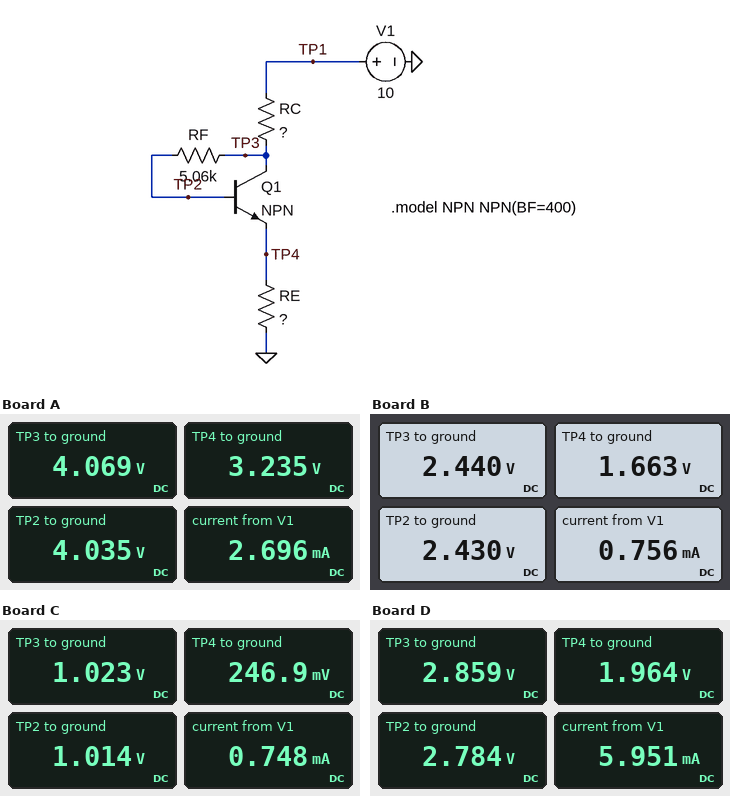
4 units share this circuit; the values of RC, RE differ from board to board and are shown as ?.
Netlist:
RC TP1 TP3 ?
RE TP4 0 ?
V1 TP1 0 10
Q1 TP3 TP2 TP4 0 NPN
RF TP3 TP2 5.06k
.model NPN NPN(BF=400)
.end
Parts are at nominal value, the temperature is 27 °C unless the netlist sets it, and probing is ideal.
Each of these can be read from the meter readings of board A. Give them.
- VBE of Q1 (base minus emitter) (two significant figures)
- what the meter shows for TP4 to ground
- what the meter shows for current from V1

800 mV
3.235 V
2.696 mA
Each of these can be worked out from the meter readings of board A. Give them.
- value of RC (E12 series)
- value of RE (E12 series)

2.2 kΩ
1.2 kΩ
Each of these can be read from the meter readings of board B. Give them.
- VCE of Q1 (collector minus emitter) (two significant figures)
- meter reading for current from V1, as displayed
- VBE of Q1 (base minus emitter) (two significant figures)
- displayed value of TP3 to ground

780 mV
0.756 mA
770 mV
2.440 V
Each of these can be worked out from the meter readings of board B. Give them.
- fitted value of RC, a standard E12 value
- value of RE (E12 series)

10 kΩ
2.2 kΩ
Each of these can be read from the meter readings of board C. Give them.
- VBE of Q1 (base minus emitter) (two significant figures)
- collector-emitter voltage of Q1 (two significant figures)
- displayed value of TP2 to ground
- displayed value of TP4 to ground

770 mV
780 mV
1.014 V
246.9 mV
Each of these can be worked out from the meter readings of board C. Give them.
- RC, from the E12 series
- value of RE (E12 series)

12 kΩ
330 Ω
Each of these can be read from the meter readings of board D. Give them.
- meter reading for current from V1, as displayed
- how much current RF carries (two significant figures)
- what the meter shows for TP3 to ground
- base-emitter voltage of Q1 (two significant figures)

5.951 mA
15 µA
2.859 V
820 mV
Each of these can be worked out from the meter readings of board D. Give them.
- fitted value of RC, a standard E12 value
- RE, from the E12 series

1.2 kΩ
330 Ω
